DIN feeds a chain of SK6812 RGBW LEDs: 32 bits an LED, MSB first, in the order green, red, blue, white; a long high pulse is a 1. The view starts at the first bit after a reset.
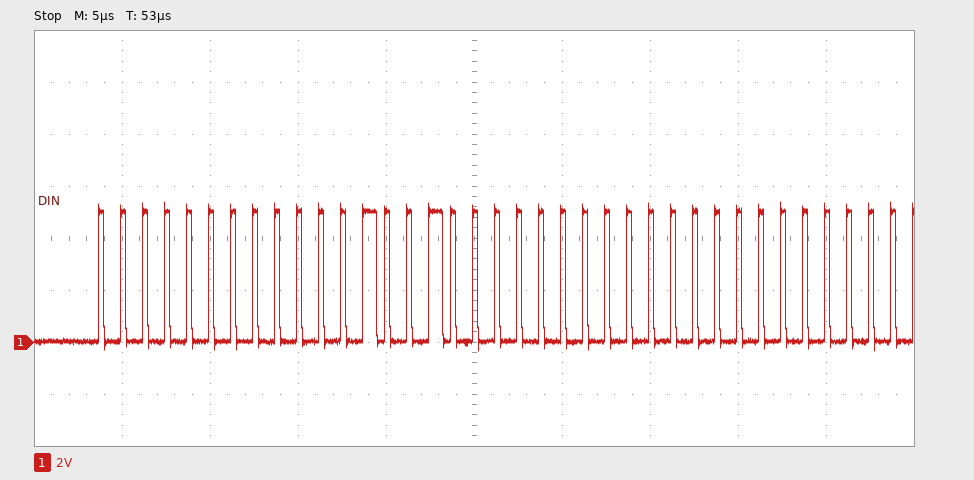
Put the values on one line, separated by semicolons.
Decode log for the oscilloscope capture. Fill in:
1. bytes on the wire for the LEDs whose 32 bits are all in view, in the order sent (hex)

00 09 00 00
